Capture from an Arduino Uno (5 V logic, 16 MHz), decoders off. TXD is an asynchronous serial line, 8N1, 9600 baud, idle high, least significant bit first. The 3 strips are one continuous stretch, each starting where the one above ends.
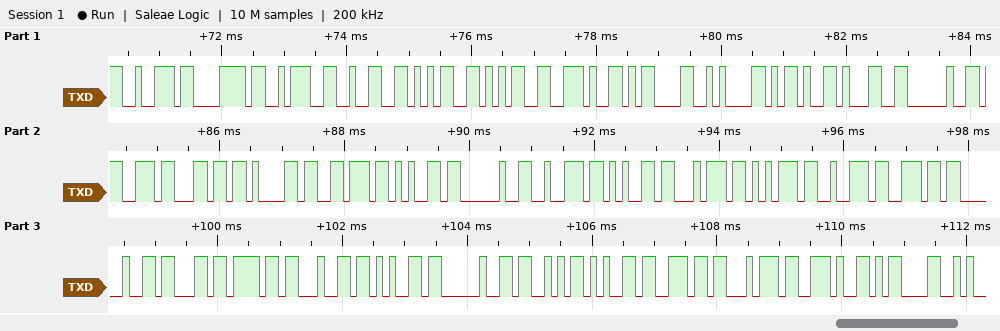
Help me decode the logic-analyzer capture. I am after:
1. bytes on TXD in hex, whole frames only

72 78 3A 32 35 35 2E 0D 0A 2D 31 20 73 6C 61 76 65 20 72 65 74 75 72 6E 20 63 6F 64 65 20 53 65 6E 74 2E 0D
